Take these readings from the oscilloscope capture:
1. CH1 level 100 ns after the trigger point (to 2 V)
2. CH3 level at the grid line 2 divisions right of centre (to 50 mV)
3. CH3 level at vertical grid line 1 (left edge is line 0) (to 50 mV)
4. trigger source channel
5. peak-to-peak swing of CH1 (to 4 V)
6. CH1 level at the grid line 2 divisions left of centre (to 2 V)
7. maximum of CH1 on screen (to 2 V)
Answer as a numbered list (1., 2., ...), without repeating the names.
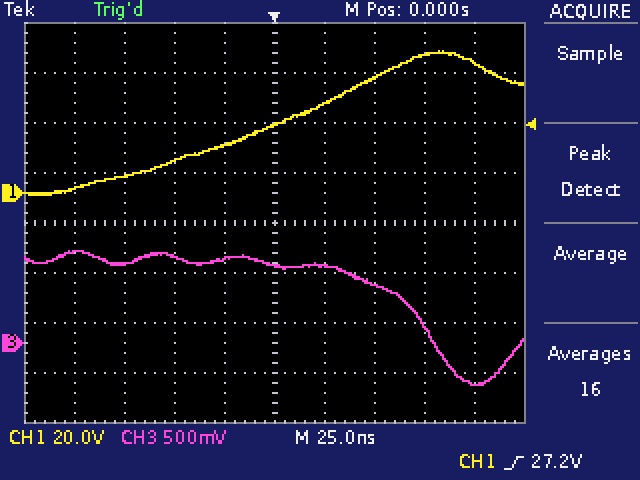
1. 52 V
2. 600 mV
3. 900 mV
4. CH1
5. 56 V
6. 12 V
7. 56 V
